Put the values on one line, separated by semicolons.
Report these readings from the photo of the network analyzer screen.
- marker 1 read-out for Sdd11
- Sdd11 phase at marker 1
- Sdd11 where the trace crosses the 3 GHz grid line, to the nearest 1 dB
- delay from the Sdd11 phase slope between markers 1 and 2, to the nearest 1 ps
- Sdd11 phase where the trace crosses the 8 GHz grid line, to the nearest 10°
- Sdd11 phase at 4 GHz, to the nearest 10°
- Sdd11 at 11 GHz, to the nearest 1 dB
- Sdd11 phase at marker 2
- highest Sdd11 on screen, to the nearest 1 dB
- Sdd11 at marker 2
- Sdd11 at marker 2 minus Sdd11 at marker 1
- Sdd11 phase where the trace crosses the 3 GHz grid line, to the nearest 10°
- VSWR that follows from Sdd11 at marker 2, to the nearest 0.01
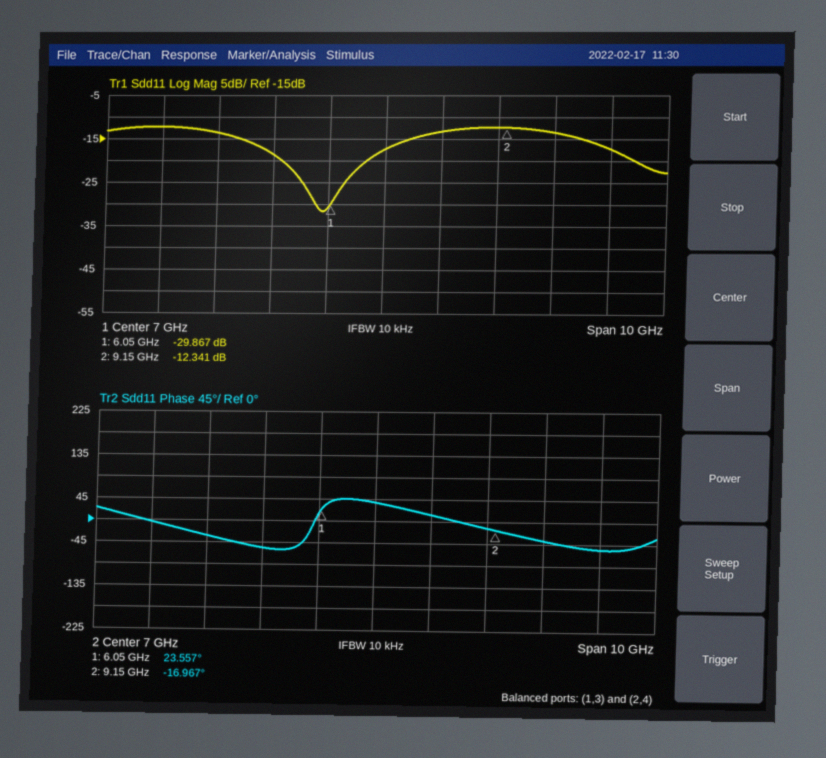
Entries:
-29.867 dB; 23.557°; -12 dB; 36 ps; 10°; -30°; -17 dB; -16.967°; -12 dB; -12.341 dB; 17.526 dB; 0°; 1.64
